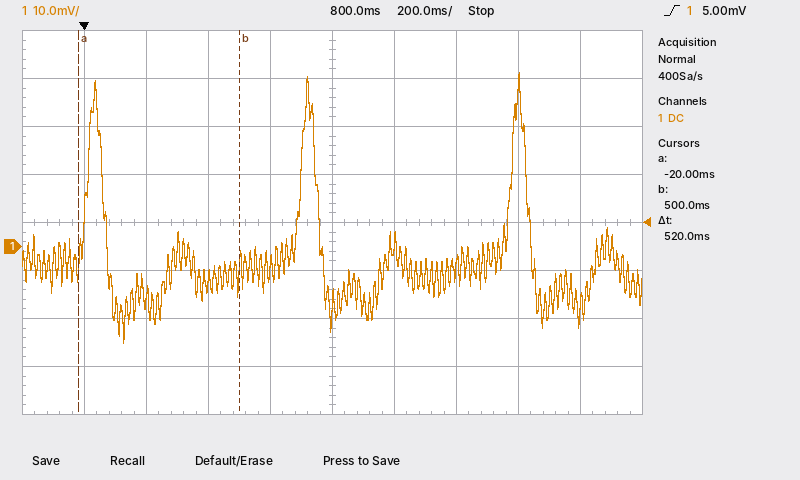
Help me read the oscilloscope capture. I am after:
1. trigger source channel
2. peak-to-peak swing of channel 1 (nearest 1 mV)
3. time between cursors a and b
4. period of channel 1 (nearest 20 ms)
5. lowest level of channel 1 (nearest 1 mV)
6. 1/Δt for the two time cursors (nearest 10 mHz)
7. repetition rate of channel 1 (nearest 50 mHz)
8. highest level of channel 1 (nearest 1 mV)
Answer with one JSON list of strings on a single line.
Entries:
["channel 1", "56 mV", "520 ms", "680 ms", "-20 mV", "1.92 Hz", "1.45 Hz", "36 mV"]
